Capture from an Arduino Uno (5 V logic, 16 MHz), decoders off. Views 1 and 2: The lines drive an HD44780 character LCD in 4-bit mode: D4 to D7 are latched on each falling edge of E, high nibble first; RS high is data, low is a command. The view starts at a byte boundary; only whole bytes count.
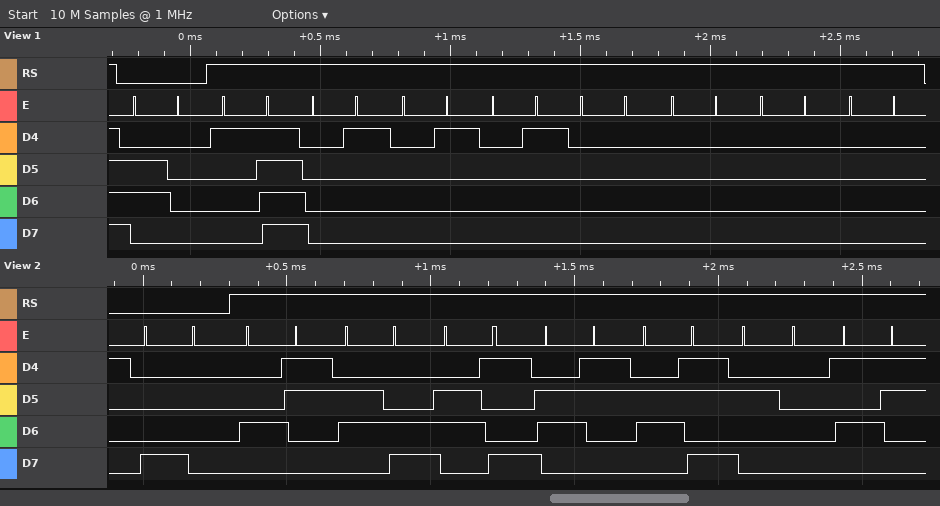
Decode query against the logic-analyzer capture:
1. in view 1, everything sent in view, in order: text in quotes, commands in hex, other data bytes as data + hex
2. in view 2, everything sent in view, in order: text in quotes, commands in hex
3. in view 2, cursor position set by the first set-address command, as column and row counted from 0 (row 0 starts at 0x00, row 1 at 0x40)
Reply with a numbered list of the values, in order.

1. 0x60 data 1F 01 01 01 00 00 00 00
2. 0x80 "Click S"
3. column 0, row 0
